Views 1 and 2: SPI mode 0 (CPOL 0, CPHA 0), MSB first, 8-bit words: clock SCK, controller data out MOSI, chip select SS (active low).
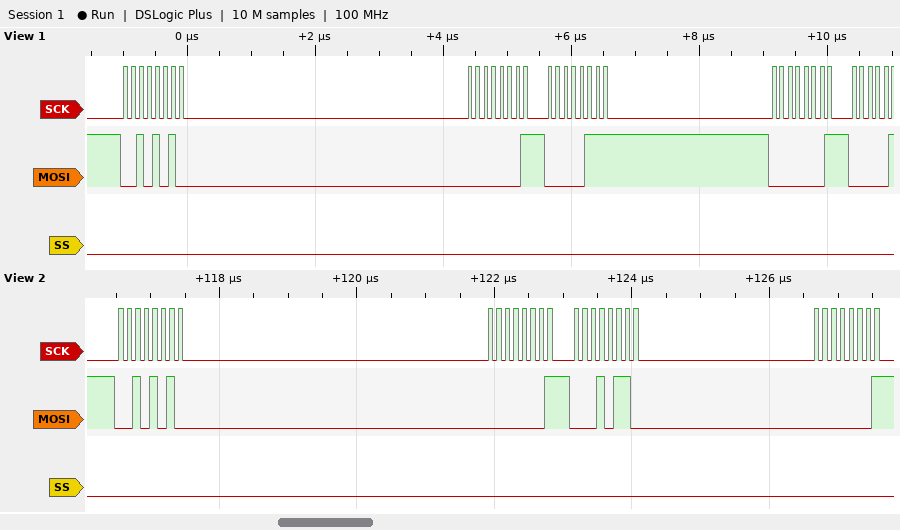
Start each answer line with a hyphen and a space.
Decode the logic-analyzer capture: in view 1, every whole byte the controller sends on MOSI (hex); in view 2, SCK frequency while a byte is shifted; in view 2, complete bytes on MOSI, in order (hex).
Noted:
- 2A 01 07 01
- 8 MHz
- 2A 01 16 01
